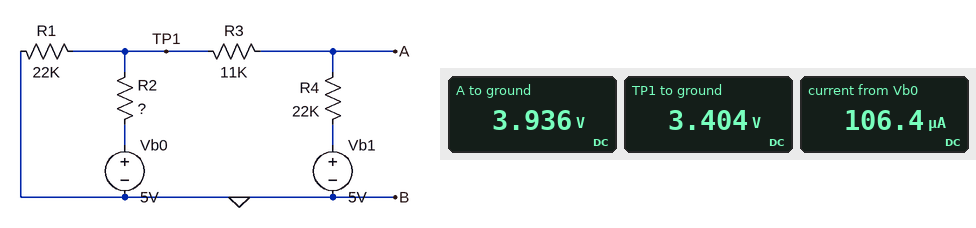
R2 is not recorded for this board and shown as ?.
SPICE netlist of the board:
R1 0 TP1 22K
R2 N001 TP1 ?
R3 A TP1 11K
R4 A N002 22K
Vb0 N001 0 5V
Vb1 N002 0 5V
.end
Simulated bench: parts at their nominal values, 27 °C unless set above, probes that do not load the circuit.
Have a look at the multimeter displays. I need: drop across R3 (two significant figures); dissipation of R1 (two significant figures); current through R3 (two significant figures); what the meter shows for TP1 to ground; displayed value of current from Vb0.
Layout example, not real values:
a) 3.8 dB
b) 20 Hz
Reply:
a) 530 mV
b) 530 µW
c) 48 µA
d) 3.404 V
e) 106.4 µA
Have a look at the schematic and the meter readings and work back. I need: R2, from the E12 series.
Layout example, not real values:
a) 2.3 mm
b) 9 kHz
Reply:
a) 15 kΩ
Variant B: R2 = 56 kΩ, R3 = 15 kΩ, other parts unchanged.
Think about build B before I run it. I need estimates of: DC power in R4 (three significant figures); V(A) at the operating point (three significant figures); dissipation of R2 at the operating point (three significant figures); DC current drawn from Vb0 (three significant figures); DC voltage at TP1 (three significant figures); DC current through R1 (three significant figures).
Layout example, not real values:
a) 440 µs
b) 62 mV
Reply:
a) 102 µW
b) 3.50 V
c) 113 µW
d) 44.9 µA
e) 2.48 V
f) 113 µA
